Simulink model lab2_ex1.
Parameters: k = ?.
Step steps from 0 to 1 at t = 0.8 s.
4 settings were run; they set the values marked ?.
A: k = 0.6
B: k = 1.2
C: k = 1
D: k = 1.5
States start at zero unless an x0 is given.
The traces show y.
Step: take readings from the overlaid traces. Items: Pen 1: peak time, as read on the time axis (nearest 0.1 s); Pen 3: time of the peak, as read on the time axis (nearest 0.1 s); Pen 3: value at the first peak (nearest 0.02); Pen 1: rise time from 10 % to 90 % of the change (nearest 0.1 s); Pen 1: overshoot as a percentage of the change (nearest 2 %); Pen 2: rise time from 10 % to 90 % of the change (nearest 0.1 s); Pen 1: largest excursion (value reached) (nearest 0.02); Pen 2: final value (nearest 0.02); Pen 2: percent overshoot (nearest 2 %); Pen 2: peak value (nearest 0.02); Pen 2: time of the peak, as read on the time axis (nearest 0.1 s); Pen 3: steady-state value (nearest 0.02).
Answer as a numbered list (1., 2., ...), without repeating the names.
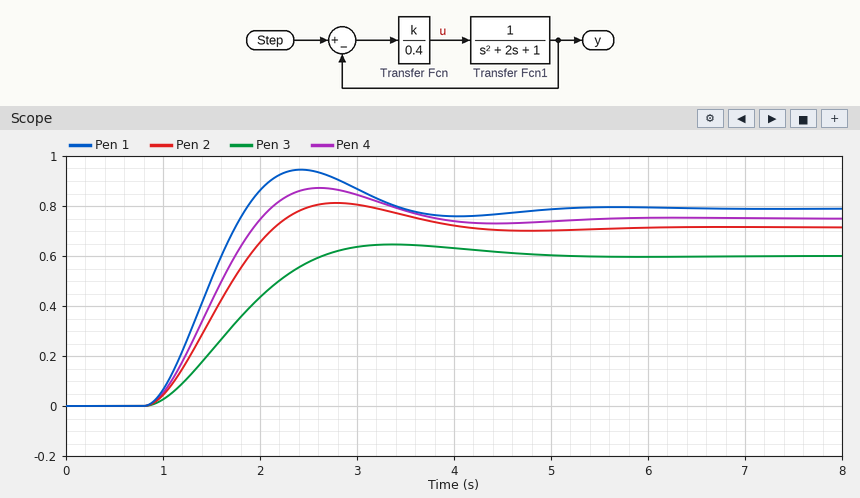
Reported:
1. 2.4 s
2. 3.4 s
3. 0.64
4. 0.7 s
5. 20 %
6. 0.9 s
7. 0.94
8. 0.72
9. 14 %
10. 0.82
11. 2.8 s
12. 0.60
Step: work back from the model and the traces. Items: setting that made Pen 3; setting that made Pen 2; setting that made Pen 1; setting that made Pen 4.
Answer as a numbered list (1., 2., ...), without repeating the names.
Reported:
1. A
2. C
3. D
4. B
